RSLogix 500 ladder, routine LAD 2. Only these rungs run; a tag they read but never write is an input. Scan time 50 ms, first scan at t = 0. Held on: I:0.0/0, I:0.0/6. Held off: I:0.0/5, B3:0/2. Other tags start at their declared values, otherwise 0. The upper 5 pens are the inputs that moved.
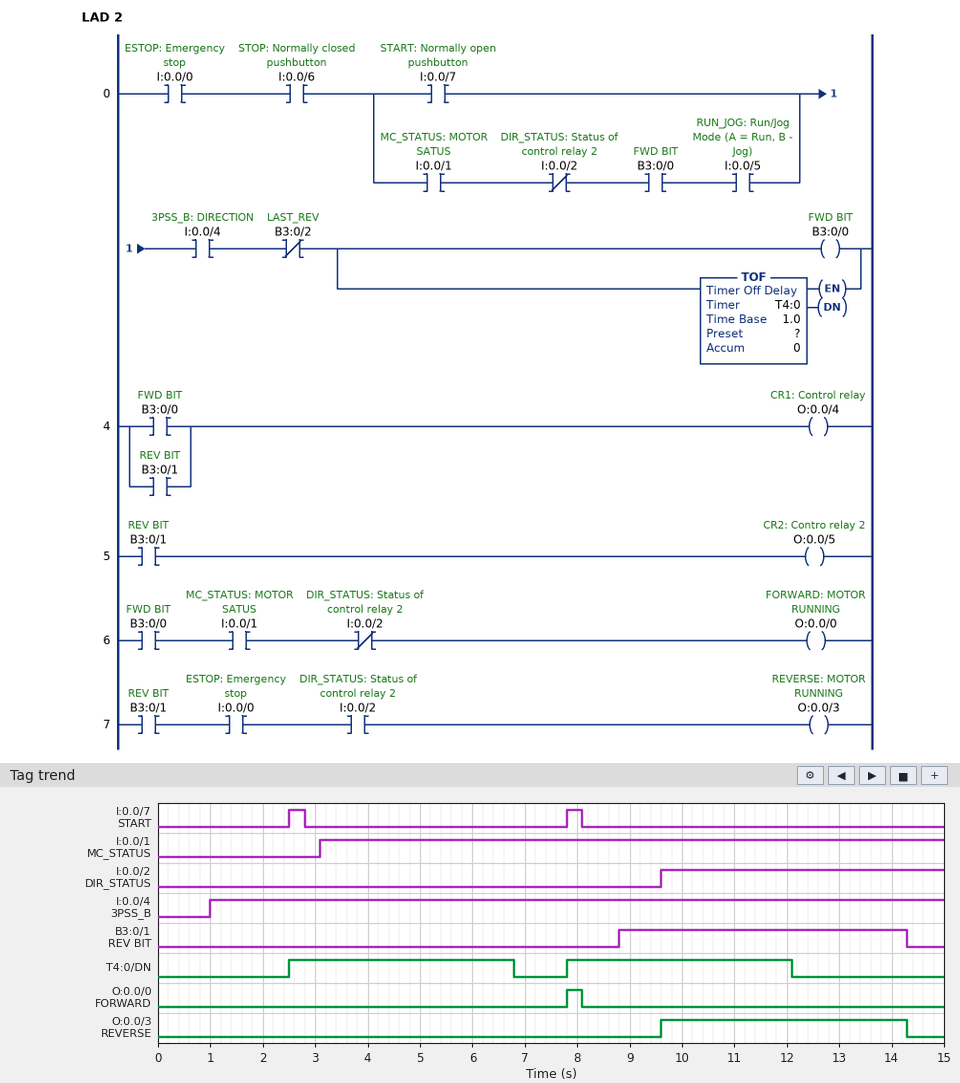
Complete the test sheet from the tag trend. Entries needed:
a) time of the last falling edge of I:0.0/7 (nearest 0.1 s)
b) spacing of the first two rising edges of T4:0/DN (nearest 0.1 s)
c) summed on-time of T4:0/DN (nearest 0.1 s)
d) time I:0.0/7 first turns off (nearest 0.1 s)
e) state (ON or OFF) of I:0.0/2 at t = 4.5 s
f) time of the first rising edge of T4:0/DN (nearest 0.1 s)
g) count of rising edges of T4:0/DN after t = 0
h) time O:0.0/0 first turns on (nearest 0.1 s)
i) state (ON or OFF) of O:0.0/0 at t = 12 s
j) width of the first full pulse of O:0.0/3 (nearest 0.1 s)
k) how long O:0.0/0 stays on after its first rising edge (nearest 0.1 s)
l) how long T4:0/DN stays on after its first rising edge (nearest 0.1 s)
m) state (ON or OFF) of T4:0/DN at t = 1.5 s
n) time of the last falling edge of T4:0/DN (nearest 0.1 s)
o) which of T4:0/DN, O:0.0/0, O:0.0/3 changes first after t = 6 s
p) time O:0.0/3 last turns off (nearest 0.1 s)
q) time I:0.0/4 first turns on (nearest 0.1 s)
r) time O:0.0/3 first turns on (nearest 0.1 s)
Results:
8.1 s
5.3 s
8.6 s
2.8 s
OFF
2.5 s
2
7.8 s
OFF
4.7 s
0.3 s
4.3 s
OFF
12.1 s
T4:0/DN
14.3 s
1.0 s
9.6 s
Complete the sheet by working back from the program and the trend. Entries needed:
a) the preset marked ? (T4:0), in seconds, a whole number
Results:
4 s
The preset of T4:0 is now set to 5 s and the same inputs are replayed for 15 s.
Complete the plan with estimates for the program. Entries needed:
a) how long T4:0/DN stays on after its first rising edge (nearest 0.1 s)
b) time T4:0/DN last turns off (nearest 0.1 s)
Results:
10.6 s
13.1 s
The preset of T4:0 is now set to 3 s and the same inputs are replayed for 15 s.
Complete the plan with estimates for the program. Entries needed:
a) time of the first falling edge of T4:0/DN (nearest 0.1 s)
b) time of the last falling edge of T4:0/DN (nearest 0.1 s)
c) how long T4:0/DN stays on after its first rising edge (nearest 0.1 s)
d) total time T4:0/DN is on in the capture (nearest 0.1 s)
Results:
5.8 s
11.1 s
3.3 s
6.6 s
